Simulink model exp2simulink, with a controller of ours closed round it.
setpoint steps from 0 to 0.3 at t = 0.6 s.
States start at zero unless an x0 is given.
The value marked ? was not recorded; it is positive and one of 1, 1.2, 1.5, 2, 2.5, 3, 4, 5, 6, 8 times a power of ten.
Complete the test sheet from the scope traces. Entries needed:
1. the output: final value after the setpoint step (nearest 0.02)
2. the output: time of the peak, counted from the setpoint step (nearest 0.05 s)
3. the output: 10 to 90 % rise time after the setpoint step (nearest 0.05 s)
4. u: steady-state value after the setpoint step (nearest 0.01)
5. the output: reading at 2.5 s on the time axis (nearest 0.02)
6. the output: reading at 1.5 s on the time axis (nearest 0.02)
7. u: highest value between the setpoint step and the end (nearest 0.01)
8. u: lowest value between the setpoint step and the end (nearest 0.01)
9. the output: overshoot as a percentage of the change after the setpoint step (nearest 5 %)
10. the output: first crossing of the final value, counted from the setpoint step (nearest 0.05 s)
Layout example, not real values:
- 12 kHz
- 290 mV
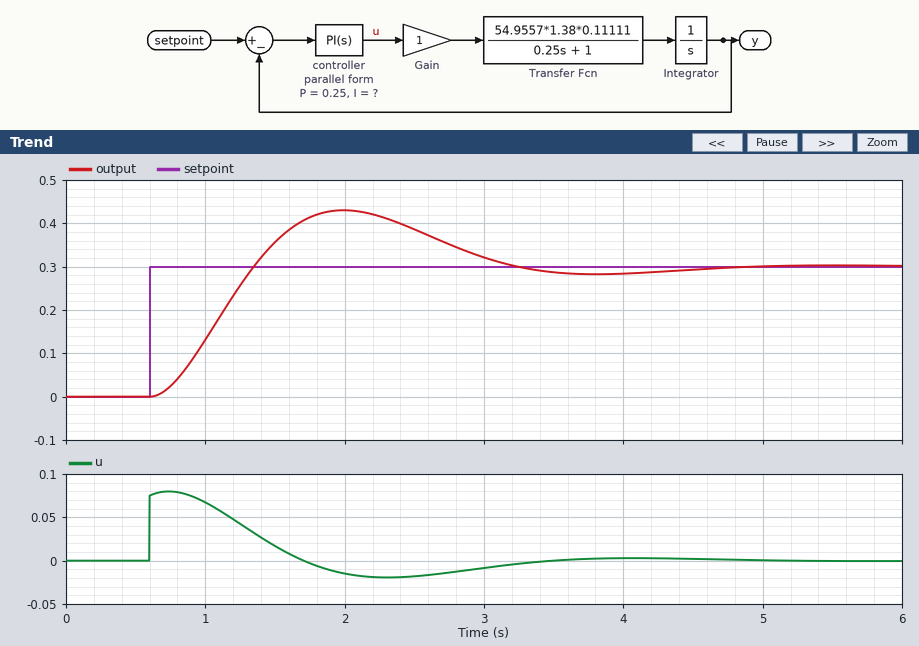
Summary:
- 0.30
- 1.40 s
- 0.50 s
- 0.00
- 0.38
- 0.36
- 0.08
- -0.02
- 45 %
- 0.75 s
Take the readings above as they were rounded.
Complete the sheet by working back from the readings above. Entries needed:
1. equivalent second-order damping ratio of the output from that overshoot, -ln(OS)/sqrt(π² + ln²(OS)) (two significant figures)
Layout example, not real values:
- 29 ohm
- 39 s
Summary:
- 0.25
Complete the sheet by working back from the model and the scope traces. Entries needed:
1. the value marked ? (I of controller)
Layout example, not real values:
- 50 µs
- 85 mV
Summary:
- 0.25
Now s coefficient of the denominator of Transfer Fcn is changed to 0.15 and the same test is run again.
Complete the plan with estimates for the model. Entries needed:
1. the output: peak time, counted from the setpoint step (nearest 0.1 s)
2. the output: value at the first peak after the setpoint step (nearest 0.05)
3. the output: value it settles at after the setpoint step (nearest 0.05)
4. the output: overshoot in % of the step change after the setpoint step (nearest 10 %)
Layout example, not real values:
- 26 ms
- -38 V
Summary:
- 1.3 s
- 0.40
- 0.30
- 30 %
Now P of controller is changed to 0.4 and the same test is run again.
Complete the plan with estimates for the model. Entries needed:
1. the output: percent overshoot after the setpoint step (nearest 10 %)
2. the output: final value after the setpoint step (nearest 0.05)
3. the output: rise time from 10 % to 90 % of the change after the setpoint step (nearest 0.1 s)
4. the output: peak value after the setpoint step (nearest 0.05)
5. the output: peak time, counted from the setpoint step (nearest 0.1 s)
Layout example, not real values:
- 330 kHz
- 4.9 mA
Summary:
- 30 %
- 0.30
- 0.4 s
- 0.40
- 1.0 s
